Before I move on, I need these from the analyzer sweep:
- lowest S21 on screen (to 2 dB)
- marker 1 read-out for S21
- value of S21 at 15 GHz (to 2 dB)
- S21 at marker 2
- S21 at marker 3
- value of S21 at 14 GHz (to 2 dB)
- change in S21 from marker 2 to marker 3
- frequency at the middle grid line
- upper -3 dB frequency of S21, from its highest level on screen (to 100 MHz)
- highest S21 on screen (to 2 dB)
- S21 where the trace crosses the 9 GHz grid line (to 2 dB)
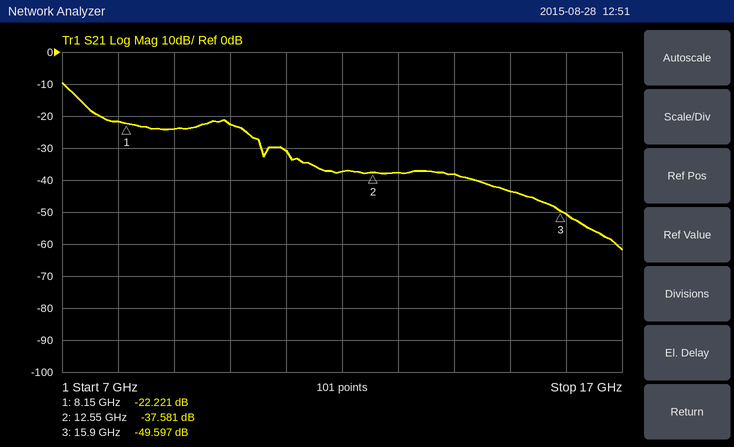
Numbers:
-62 dB
-22.221 dB
-44 dB
-37.581 dB
-49.597 dB
-38 dB
-12.016 dB
12 GHz
7.2 GHz
-10 dB
-24 dB
